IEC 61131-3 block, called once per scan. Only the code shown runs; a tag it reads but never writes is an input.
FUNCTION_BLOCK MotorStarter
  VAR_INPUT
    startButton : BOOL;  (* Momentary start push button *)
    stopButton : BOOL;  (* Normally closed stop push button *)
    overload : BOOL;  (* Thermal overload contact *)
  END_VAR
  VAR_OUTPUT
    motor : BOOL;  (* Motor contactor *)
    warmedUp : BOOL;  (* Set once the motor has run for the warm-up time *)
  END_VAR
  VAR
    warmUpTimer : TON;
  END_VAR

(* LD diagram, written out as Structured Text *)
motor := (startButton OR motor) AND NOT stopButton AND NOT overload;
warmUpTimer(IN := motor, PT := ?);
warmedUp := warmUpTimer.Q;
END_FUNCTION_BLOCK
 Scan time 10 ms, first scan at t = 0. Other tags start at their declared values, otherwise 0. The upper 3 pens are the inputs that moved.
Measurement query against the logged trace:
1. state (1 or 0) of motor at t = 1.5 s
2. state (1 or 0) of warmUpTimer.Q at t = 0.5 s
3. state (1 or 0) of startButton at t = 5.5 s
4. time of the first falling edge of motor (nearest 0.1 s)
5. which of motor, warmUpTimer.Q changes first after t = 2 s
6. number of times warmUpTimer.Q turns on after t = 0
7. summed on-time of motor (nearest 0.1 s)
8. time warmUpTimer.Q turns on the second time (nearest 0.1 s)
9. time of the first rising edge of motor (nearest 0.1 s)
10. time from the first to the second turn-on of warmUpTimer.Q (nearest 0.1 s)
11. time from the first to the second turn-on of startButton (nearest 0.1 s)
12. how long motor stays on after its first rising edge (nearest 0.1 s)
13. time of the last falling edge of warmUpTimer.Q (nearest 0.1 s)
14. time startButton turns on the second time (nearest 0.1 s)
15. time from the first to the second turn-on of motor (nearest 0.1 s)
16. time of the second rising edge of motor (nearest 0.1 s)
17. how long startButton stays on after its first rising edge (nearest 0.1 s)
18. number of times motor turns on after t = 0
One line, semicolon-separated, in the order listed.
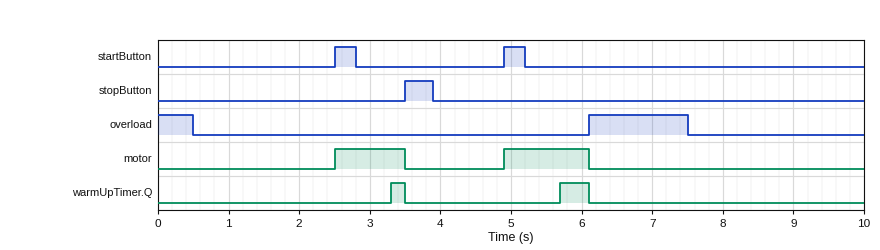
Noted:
0; 0; 0; 3.5 s; motor; 2; 2.2 s; 5.7 s; 2.5 s; 2.4 s; 2.4 s; 1.0 s; 6.1 s; 4.9 s; 2.4 s; 4.9 s; 0.3 s; 2
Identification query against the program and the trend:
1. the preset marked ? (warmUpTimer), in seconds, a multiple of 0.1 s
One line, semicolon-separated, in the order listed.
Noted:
0.8 s
